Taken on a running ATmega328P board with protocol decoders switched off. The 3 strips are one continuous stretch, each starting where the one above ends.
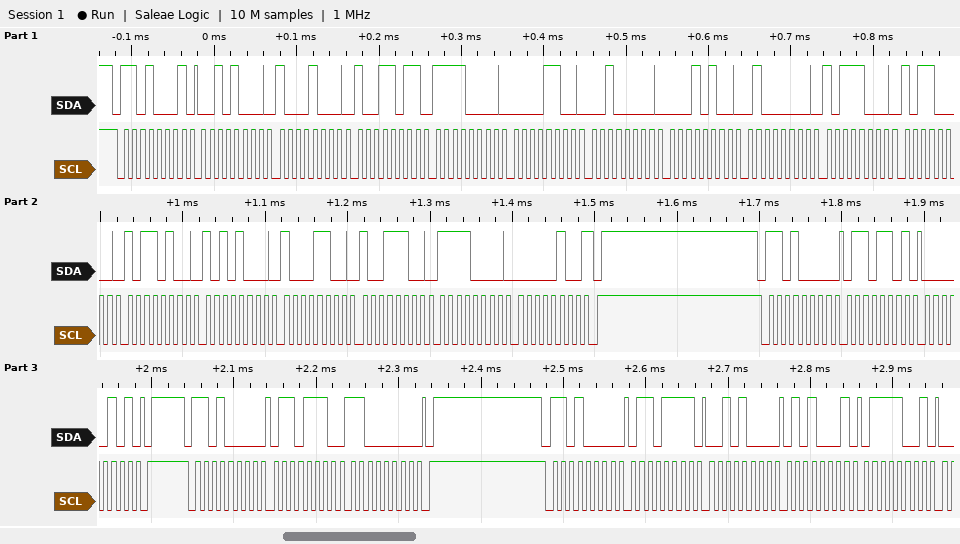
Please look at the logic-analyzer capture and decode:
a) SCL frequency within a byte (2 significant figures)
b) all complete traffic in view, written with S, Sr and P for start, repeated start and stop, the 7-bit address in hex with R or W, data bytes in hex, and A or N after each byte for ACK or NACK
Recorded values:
100 kHz
S 68R A 28 A 88 A 9B A F0 A 0C A 20 A 14 A 40 A B8 A B0 A B4 A A8 A 8C A 9C A F0 A 04 N P S 68W A 6D A 05 A P S 68W A 6E A C0 A P S 68W A 6F A 28 A 51 A 79 A
